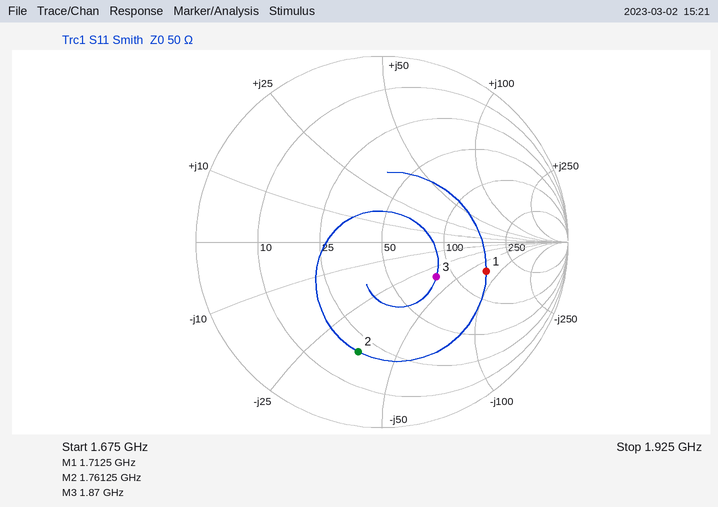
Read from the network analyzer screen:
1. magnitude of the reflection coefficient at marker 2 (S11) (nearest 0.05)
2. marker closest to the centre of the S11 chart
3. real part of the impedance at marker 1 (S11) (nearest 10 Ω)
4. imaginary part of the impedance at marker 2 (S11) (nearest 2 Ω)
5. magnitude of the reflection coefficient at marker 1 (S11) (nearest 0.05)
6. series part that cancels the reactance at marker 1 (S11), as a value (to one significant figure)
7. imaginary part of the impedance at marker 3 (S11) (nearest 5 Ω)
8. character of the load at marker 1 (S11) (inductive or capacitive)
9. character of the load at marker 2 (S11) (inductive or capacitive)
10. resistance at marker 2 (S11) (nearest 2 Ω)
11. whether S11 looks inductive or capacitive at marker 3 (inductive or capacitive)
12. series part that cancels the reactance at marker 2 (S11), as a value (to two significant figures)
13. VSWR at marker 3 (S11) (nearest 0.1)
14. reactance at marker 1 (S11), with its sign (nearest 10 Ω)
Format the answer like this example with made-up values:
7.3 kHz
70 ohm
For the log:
0.60
marker 3
150 Ω
-36 Ω
0.60
7 nH
-35 Ω
capacitive
capacitive
20 Ω
capacitive
3.3 nH
2.1
-70 Ω
